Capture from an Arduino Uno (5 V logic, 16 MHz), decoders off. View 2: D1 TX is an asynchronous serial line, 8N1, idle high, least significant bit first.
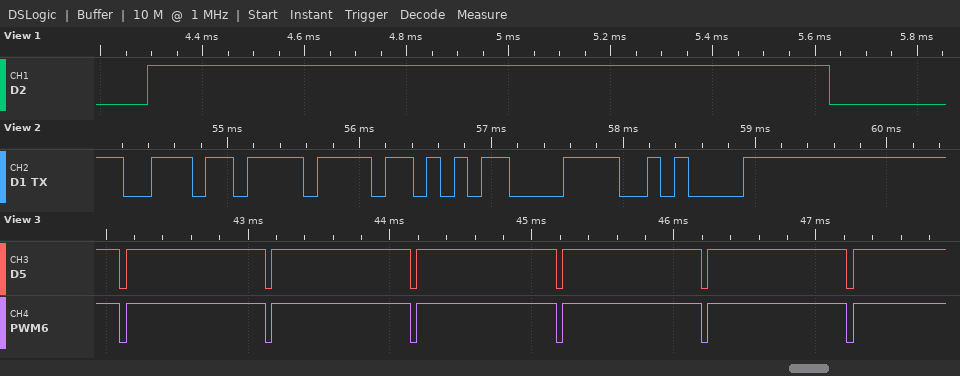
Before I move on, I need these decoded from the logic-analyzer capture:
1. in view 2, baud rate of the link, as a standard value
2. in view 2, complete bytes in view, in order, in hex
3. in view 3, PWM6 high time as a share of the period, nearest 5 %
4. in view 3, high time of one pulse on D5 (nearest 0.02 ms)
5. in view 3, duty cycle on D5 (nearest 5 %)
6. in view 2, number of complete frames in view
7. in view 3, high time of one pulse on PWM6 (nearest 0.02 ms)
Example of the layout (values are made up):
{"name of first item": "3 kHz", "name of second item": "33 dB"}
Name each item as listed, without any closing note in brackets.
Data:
{"in view 2, baud rate of the link, as a standard value": "9600 baud", "in view 2, complete bytes in view, in order, in hex": "6E 6F 0D 0A", "in view 3, PWM6 high time as a share of the period, nearest 5 %": "95 %", "in view 3, high time of one pulse on D5": "0.98 ms", "in view 3, duty cycle on D5": "95 %", "in view 2, number of complete frames in view": "4", "in view 3, high time of one pulse on PWM6": "0.98 ms"}
